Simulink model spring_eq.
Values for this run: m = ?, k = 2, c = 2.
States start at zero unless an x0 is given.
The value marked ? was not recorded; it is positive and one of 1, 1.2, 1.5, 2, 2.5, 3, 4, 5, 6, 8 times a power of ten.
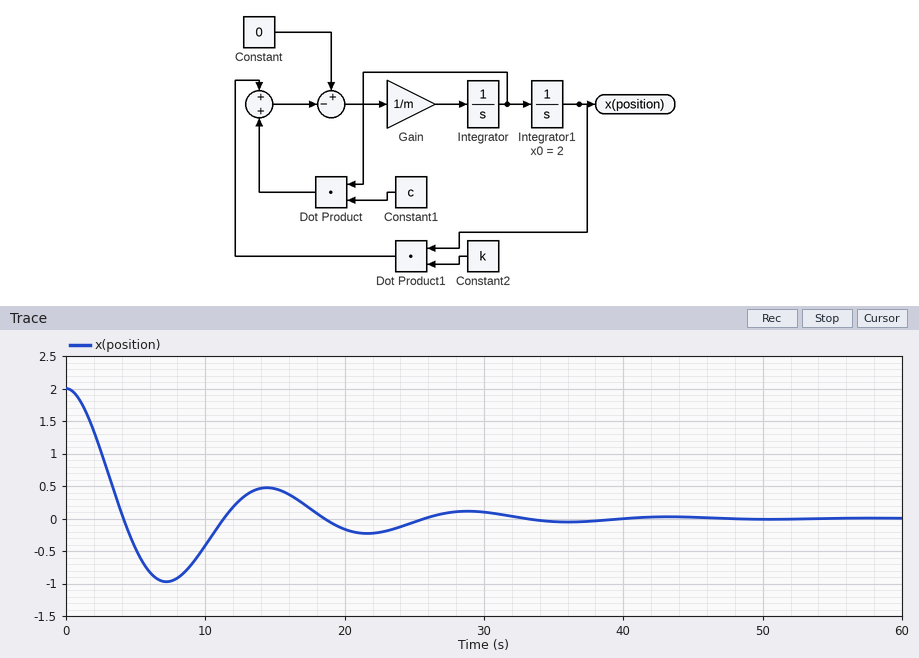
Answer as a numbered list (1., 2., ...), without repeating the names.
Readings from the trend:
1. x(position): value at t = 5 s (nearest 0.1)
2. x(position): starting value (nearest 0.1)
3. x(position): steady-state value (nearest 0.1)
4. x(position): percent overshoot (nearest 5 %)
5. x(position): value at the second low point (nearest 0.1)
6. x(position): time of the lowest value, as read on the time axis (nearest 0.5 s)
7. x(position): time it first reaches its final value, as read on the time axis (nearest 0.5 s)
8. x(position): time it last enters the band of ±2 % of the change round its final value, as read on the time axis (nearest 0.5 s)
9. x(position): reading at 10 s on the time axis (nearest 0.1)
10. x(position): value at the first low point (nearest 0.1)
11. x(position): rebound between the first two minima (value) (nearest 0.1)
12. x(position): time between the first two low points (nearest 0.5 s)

1. -0.5
2. 2.0
3. 0.0
4. 50 %
5. -0.2
6. 7.0 s
7. 4.0 s
8. 38.0 s
9. -0.4
10. -1.0
11. 0.5
12. 14.5 s
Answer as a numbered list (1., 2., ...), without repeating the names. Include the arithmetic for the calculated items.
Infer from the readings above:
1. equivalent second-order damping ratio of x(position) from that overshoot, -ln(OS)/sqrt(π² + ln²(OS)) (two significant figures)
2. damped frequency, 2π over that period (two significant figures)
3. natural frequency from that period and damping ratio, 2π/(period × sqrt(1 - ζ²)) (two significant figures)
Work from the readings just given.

1. ln(0.5) = -0.693; 0.693 / sqrt(9.870 + 0.480) = 0.22
2. 2π / 14.5 = 0.43 rad/s
3. 2π / (14.5 × sqrt(1 - 0.22²)) = 0.44 rad/s
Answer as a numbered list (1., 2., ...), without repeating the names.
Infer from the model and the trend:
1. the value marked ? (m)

1. 10
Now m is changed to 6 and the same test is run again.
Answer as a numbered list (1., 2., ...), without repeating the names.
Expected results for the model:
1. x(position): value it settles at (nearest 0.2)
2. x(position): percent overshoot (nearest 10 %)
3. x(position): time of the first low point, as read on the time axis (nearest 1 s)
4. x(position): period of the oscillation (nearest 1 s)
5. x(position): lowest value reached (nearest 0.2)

1. 0.0
2. 40 %
3. 6 s
4. 11 s
5. -0.8
